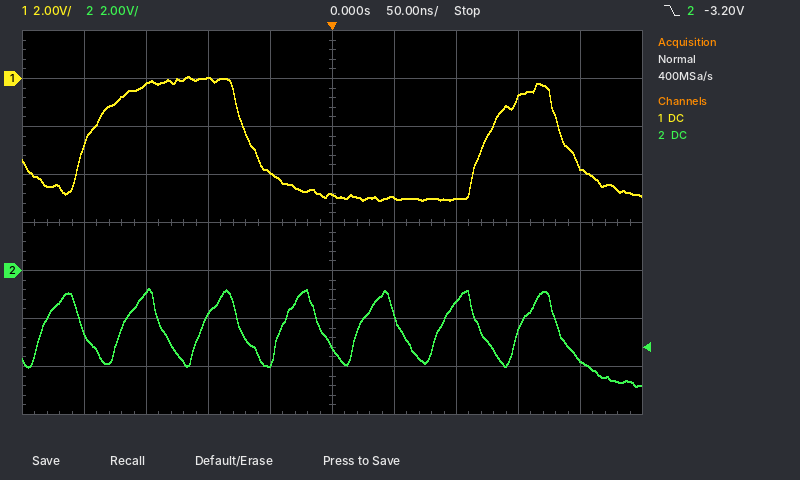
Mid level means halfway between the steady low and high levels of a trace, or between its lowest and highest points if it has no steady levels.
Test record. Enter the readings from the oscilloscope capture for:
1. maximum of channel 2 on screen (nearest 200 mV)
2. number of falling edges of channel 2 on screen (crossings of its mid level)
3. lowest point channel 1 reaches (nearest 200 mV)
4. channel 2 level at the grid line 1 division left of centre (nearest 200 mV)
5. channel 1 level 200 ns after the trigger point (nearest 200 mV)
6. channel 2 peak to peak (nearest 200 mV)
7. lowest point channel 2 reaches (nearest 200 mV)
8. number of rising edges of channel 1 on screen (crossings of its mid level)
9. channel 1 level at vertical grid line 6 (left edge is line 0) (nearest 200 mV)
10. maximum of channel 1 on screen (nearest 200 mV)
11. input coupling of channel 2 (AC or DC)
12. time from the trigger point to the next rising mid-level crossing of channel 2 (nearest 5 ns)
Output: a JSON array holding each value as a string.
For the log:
["-800 mV", "7", "-5.0 V", "-3.8 V", "-3.6 V", "4.0 V", "-4.8 V", "2", "-5.0 V", "0.0 V", "DC", "20 ns"]
